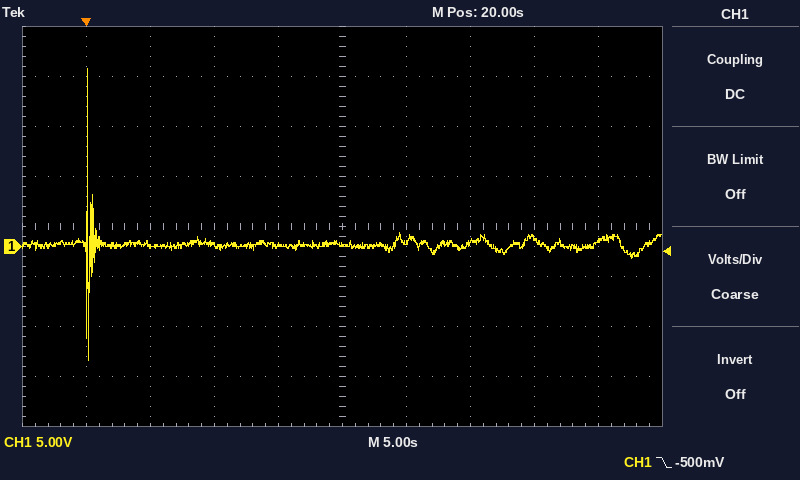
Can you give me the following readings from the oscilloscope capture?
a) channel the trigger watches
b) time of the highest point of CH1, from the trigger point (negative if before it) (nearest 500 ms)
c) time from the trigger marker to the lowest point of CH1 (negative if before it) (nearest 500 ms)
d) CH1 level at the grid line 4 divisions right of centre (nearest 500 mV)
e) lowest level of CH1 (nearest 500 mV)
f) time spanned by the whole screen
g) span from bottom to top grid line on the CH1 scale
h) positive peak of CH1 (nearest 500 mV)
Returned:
CH1
0.0 s
0.0 s
500 mV
-11.5 V
50 s
40 V
18.0 V
